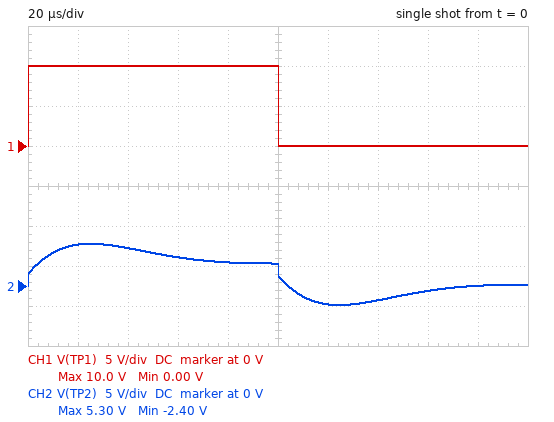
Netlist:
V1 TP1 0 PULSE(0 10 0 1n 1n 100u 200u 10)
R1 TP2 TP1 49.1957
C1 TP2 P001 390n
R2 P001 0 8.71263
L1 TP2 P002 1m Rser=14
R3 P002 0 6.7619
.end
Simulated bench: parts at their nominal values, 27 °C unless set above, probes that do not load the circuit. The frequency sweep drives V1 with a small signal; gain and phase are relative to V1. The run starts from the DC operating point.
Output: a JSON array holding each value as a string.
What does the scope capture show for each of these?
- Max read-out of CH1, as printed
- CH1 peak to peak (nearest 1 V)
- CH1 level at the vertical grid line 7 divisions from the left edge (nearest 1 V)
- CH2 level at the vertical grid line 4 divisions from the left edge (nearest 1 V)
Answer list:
["10.0 V", "10 V", "0 V", "3 V"]
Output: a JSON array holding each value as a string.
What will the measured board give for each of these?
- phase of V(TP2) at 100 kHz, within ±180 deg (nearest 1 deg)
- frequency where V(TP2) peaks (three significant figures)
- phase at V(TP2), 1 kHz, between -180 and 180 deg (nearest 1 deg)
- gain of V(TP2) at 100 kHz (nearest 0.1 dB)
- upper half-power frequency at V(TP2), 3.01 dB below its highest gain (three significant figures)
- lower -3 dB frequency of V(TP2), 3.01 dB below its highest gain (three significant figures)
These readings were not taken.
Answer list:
["-20 deg", "8.49 kHz", "10 deg", "-15.6 dB", "16.2 kHz", "3.97 kHz"]
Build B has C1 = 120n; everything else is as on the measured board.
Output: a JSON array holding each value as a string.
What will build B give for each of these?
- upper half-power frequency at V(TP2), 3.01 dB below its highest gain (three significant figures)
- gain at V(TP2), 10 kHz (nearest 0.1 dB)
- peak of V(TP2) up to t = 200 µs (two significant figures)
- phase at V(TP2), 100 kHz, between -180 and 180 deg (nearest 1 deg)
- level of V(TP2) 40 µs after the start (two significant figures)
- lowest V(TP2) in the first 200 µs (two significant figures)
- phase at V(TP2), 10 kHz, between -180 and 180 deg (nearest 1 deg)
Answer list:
["34.9 kHz", "-2.3 dB", "6.9 V", "-43 deg", "3.6 V", "-3.9 V", "15 deg"]
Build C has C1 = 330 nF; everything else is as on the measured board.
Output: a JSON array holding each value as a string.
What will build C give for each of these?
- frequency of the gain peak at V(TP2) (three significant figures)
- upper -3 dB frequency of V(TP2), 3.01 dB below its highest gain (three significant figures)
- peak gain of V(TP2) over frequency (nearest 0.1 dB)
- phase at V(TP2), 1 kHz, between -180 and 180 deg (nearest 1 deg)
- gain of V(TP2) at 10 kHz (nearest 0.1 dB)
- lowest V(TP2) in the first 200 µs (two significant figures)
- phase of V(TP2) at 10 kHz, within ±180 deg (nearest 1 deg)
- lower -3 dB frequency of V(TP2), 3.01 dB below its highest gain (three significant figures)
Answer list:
["9.27 kHz", "17.9 kHz", "-3.1 dB", "10 deg", "-3.2 dB", "-2.6 V", "-11 deg", "4.36 kHz"]
